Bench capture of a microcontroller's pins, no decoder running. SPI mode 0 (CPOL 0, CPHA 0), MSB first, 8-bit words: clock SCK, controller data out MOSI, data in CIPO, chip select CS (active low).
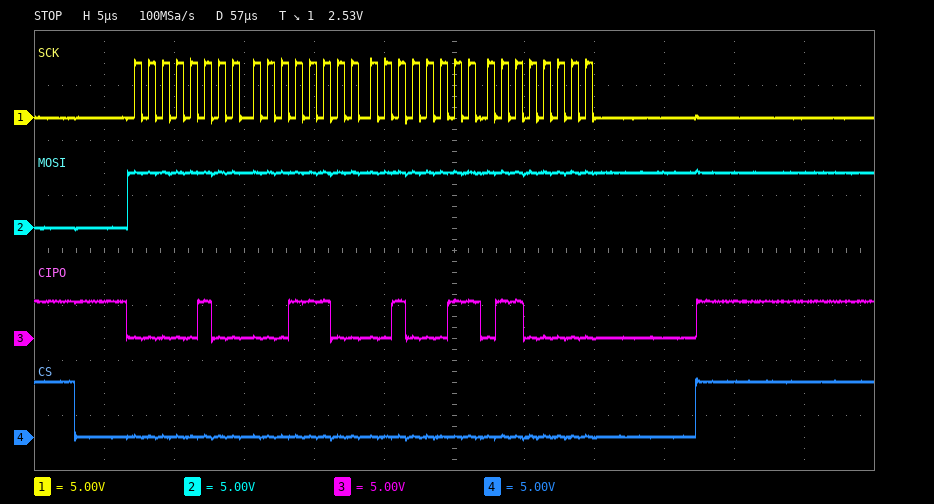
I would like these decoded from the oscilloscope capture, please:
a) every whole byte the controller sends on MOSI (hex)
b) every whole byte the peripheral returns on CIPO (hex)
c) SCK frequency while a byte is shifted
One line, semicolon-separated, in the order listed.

FF FF FF FF; 04 1C 23 60; 1 MHz
